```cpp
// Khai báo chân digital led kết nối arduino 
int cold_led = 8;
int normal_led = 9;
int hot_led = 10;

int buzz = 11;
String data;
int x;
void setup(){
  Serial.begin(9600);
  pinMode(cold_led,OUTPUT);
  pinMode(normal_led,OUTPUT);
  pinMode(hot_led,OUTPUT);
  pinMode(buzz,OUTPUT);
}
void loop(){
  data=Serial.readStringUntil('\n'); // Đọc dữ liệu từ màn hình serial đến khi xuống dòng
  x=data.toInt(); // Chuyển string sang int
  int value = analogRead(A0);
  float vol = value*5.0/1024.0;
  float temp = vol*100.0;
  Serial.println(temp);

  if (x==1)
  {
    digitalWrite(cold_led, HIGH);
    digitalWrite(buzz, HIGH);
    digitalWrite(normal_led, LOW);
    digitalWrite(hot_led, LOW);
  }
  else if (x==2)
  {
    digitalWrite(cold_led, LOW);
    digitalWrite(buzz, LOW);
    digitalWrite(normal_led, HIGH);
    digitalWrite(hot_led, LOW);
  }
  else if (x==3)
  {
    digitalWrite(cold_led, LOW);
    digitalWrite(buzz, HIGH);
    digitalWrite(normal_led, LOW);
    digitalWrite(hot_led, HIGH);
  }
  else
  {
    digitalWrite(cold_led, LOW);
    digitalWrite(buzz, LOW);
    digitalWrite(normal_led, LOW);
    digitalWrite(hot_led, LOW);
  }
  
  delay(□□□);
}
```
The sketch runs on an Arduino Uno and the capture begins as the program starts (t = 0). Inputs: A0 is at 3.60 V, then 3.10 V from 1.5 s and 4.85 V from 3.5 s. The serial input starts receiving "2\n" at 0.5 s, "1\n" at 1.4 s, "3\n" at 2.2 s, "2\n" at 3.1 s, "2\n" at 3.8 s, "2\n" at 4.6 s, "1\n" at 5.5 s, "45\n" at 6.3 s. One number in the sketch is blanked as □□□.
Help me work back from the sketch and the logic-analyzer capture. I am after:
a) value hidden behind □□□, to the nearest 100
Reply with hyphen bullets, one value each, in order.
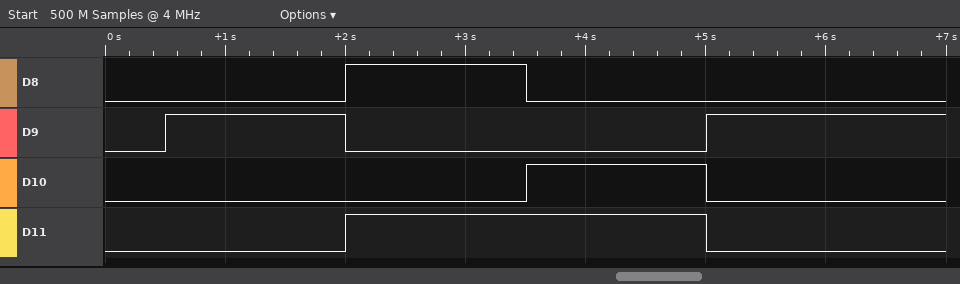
- 1500
